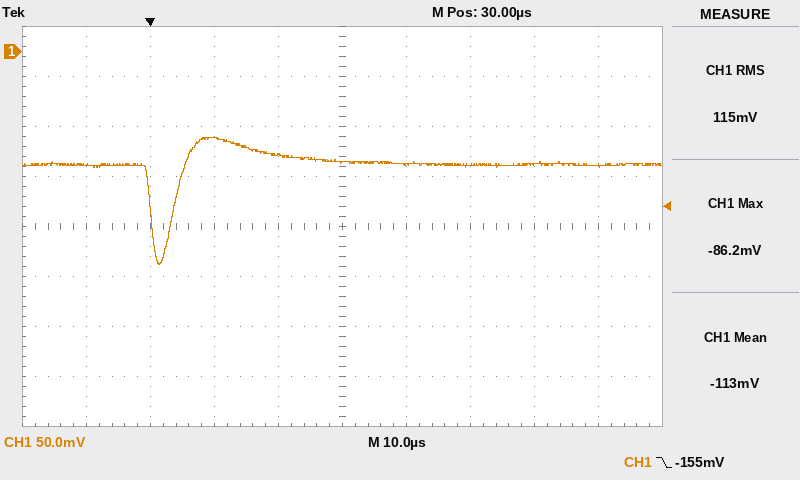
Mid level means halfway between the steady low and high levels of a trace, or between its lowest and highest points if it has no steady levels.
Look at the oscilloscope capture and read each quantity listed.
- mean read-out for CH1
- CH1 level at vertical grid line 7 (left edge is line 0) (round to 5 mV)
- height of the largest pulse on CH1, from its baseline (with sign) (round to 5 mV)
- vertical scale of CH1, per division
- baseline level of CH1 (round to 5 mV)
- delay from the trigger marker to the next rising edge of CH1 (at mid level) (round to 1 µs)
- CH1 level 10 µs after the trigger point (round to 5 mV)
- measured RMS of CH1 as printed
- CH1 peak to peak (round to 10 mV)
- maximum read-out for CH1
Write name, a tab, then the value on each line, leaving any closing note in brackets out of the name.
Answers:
mean read-out for CH1	-113 mV
CH1 level at vertical grid line 7 (left edge is line 0)	-115 mV
height of the largest pulse on CH1, from its baseline (with sign)	-100 mV
vertical scale of CH1, per division	50 mV
baseline level of CH1	-115 mV
delay from the trigger marker to the next rising edge of CH1 (at mid level)	4 µs
CH1 level 10 µs after the trigger point	-85 mV
measured RMS of CH1 as printed	115 mV
CH1 peak to peak	130 mV
maximum read-out for CH1	-86.2 mV
